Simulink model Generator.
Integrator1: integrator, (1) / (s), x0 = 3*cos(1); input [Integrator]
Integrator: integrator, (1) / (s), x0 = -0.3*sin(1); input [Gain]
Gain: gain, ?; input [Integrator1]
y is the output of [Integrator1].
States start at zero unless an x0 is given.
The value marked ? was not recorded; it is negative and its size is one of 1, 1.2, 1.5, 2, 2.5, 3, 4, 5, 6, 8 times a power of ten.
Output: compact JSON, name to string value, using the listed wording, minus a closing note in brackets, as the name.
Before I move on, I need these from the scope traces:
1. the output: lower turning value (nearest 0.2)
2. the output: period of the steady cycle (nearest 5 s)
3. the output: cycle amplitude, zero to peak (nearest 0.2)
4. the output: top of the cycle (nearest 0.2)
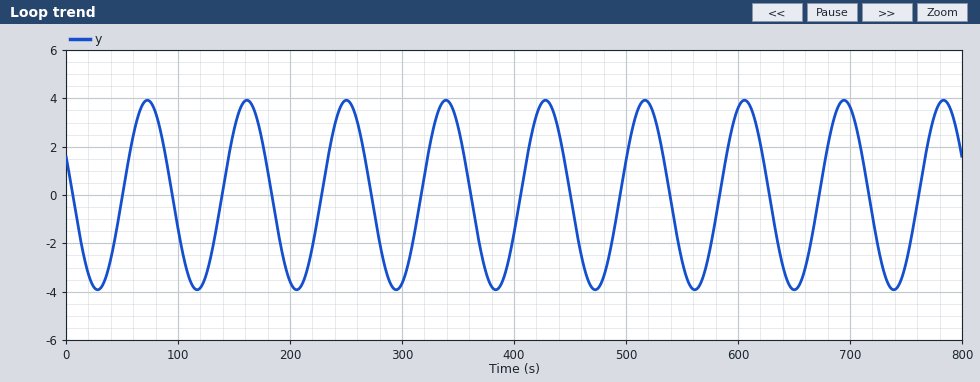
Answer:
{"the output: lower turning value": "-4.0", "the output: period of the steady cycle": "90 s", "the output: cycle amplitude, zero to peak": "4.0", "the output: top of the cycle": "4.0"}
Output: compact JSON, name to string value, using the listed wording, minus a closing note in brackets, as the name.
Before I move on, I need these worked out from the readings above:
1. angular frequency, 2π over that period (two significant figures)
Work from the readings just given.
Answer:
{"angular frequency, 2π over that period": "0.070 rad/s"}
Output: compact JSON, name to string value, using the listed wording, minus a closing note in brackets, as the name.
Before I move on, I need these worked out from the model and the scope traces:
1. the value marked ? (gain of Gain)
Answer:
{"the value marked ?": "-0.005"}
